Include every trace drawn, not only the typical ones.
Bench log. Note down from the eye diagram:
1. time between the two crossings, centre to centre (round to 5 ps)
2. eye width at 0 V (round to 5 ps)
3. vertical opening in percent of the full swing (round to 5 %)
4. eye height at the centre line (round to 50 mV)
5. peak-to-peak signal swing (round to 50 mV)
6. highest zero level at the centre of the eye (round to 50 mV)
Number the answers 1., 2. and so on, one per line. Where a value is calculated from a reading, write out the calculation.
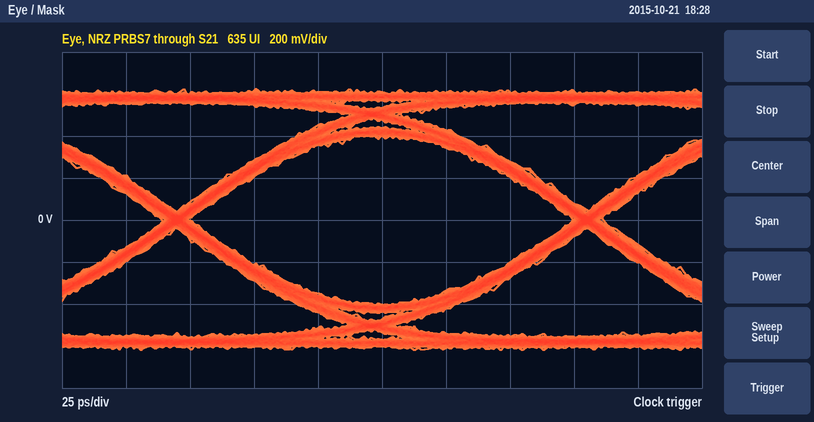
1. 160 ps
2. 150 ps
3. 800 mV / 1.25 V ≈ 64.0 %, so 65 % to the nearest 5 %
4. 800 mV
5. 1.25 V
6. -400 mV
